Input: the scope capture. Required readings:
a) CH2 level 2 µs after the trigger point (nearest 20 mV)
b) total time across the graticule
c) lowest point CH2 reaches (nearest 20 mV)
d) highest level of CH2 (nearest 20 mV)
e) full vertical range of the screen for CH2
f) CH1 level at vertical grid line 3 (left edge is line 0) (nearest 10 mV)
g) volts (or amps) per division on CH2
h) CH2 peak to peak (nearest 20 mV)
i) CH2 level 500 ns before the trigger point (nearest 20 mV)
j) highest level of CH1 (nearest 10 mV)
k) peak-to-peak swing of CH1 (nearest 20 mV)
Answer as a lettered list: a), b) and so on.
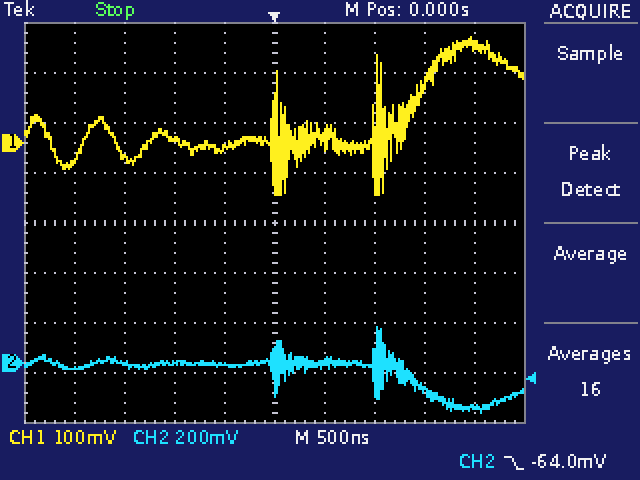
a) -180 mV
b) 5 µs
c) -200 mV
d) 140 mV
e) 1.6 V
f) 10 mV
g) 200 mV
h) 340 mV
i) 0 mV
j) 210 mV
k) 320 mV
